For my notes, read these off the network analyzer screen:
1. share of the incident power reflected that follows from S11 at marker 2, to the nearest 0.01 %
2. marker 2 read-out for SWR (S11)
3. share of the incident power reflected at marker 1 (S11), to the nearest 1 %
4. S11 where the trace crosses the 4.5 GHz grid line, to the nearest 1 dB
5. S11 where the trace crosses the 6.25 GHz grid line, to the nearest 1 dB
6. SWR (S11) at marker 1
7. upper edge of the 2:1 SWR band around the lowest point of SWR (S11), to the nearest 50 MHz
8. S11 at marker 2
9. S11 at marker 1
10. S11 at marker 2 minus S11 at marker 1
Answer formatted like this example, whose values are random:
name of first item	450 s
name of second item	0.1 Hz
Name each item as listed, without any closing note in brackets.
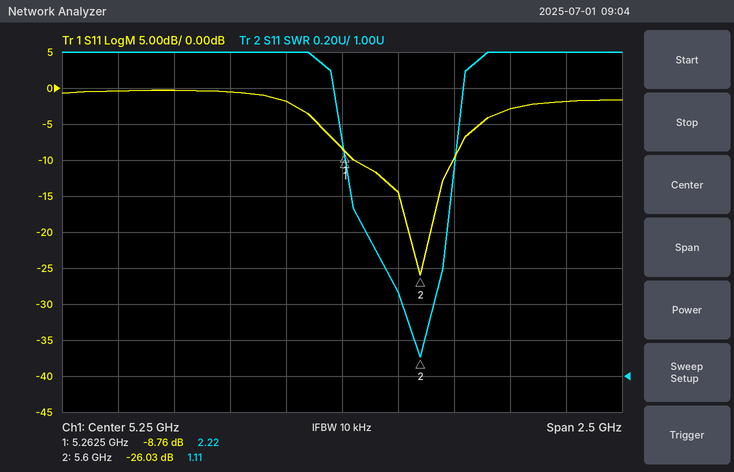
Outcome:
share of the incident power reflected that follows from S11 at marker 2, to the nearest 0.01 %	0.25 %
marker 2 read-out for SWR	1.11
share of the incident power reflected at marker 1 (S11), to the nearest 1 %	13 %
S11 where the trace crosses the 4.5 GHz grid line, to the nearest 1 dB	0 dB
S11 where the trace crosses the 6.25 GHz grid line, to the nearest 1 dB	-2 dB
SWR (S11) at marker 1	2.22
upper edge of the 2:1 SWR band around the lowest point of SWR (S11), to the nearest 50 MHz	5.75 GHz
S11 at marker 2	-26.03 dB
S11 at marker 1	-8.76 dB
S11 at marker 2 minus S11 at marker 1	-17.27 dB
